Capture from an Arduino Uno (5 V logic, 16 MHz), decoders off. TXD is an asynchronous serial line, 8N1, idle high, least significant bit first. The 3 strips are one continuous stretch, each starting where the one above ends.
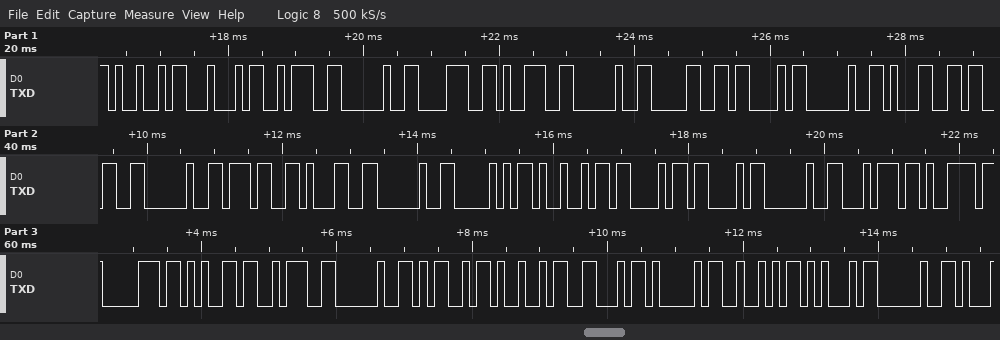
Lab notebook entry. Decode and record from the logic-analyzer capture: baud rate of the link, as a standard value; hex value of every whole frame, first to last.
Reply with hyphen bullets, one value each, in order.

- 9600 baud
- 0x49 0x44 0x3A 0x20 0x38 0x39 0x20 0x30 0x43 0x20 0x31 0x33 0x20 0x37 0x31 0x20 0x50 0x49 0x43 0x43 0x20 0x74 0x79 0x70 0x65 0x3A 0x20 0x4D 0x49 0x46 0x41 0x52 0x45 0x20
